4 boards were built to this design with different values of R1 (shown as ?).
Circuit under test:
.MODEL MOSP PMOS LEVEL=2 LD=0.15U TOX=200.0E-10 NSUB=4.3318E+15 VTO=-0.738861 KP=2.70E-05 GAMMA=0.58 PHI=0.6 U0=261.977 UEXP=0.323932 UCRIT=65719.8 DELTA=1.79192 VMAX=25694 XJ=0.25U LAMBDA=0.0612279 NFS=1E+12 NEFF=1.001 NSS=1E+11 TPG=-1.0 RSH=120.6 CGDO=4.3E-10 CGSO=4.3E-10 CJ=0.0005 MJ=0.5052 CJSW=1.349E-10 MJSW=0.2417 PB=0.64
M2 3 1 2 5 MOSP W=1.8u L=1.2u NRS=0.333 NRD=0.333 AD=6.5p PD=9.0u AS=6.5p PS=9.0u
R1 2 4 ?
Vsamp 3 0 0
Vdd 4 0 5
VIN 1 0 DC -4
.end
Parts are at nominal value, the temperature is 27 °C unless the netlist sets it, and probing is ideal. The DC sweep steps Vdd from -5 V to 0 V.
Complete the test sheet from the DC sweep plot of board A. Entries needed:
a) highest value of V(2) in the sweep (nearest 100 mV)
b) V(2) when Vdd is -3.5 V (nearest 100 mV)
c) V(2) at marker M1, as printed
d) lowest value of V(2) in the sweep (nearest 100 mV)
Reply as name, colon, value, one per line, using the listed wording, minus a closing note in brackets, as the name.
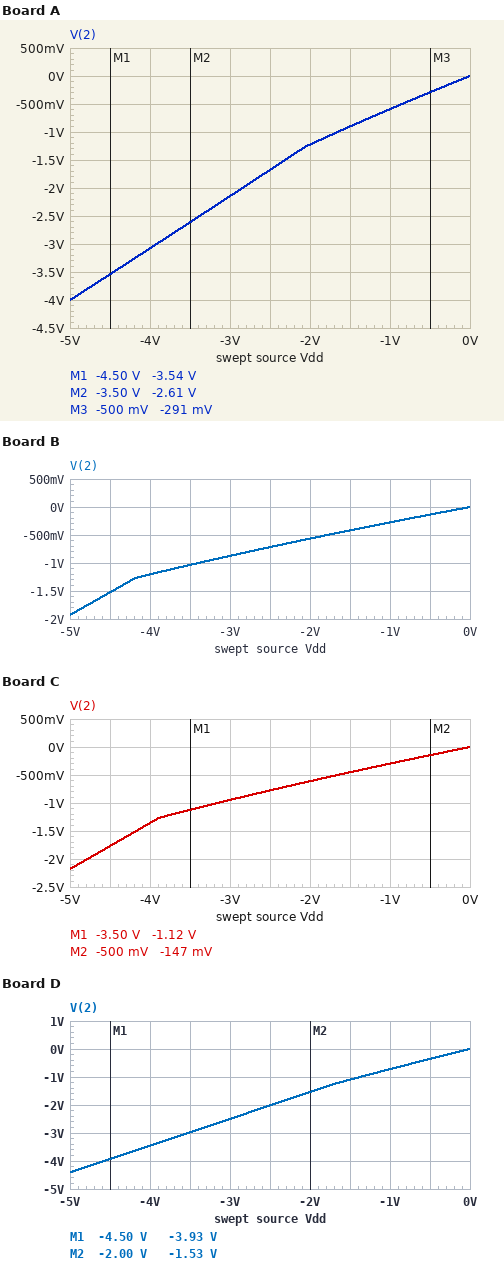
highest value of V(2) in the sweep: 0 V
V(2) when Vdd is -3.5 V: -2.6 V
V(2) at marker M1, as printed: -3.54 V
lowest value of V(2) in the sweep: -4.0 V
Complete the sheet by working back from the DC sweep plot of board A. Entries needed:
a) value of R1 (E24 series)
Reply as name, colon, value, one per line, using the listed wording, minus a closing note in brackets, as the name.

value of R1: 8.2 kΩ
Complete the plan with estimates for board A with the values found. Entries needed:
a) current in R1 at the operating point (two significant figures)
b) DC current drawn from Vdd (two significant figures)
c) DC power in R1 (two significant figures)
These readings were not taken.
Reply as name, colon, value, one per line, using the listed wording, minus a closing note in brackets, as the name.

current in R1 at the operating point: 250 µA
DC current drawn from Vdd: 250 µA
DC power in R1: 510 µW
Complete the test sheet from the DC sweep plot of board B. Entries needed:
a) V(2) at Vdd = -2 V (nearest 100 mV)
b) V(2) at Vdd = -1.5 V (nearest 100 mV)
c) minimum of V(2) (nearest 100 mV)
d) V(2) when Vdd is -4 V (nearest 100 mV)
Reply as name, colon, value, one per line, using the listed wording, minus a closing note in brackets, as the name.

V(2) at Vdd = -2 V: -600 mV
V(2) at Vdd = -1.5 V: -400 mV
minimum of V(2): -1.9 V
V(2) when Vdd is -4 V: -1.2 V
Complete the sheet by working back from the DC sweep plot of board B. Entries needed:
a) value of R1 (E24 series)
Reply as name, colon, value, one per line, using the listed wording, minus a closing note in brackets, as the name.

value of R1: 30 kΩ
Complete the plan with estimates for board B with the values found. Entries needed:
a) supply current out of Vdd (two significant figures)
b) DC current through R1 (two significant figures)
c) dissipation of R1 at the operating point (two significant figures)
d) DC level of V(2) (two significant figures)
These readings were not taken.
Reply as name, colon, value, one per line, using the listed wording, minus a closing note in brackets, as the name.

supply current out of Vdd: 130 µA
DC current through R1: 130 µA
dissipation of R1 at the operating point: 470 µW
DC level of V(2): 1.2 V
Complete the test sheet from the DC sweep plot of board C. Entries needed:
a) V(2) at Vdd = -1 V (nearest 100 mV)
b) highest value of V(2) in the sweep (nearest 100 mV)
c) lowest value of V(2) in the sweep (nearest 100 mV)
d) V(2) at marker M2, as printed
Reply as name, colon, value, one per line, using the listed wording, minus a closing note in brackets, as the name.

V(2) at Vdd = -1 V: -300 mV
highest value of V(2) in the sweep: 0 V
lowest value of V(2) in the sweep: -2.2 V
V(2) at marker M2, as printed: -147 mV
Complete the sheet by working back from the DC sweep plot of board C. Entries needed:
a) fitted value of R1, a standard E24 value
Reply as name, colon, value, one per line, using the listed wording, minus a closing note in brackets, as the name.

fitted value of R1, a standard E24 value: 27 kΩ
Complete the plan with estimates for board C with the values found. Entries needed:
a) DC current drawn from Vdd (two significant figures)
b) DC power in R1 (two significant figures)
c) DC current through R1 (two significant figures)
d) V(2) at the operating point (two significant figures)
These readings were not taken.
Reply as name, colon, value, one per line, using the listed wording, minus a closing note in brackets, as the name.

DC current drawn from Vdd: 140 µA
DC power in R1: 500 µW
DC current through R1: 140 µA
V(2) at the operating point: 1.3 V
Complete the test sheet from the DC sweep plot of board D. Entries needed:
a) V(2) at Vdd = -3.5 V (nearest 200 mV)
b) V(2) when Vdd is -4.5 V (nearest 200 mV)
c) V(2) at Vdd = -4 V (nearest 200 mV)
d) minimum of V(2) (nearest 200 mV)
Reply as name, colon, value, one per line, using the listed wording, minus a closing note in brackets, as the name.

V(2) at Vdd = -3.5 V: -3.0 V
V(2) when Vdd is -4.5 V: -4.0 V
V(2) at Vdd = -4 V: -3.4 V
minimum of V(2): -4.4 V
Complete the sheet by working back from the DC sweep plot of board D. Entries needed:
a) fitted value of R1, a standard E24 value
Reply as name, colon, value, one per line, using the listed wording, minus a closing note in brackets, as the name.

fitted value of R1, a standard E24 value: 4.7 kΩ
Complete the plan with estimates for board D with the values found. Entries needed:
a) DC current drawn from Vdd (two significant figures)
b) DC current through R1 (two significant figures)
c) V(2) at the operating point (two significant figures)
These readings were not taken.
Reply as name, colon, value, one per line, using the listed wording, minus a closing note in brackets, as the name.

DC current drawn from Vdd: 300 µA
DC current through R1: 300 µA
V(2) at the operating point: 3.6 V
